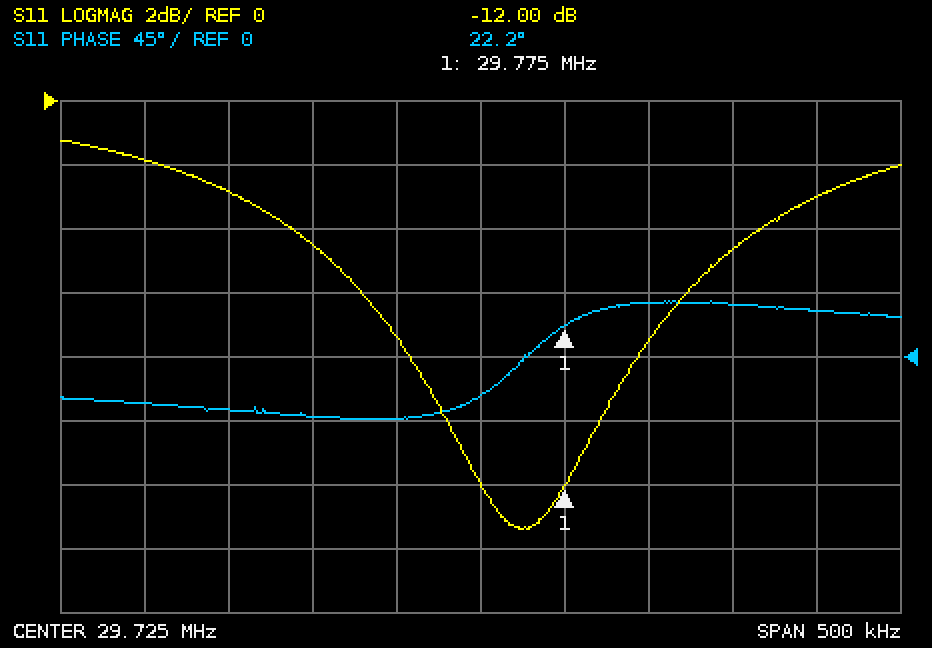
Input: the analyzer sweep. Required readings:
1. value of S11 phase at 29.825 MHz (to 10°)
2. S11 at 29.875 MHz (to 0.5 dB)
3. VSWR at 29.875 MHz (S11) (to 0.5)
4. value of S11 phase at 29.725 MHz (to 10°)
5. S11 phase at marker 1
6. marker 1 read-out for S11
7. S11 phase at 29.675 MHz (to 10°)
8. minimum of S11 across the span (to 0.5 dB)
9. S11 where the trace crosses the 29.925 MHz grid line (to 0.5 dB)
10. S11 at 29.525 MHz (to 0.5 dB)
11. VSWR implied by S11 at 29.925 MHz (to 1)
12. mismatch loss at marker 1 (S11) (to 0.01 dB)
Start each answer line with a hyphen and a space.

- 40°
- -4.5 dB
- 4.0
- -30°
- 22.2°
- -12.00 dB
- -40°
- -13.5 dB
- -3.0 dB
- -2.0 dB
- 6
- 0.28 dB
